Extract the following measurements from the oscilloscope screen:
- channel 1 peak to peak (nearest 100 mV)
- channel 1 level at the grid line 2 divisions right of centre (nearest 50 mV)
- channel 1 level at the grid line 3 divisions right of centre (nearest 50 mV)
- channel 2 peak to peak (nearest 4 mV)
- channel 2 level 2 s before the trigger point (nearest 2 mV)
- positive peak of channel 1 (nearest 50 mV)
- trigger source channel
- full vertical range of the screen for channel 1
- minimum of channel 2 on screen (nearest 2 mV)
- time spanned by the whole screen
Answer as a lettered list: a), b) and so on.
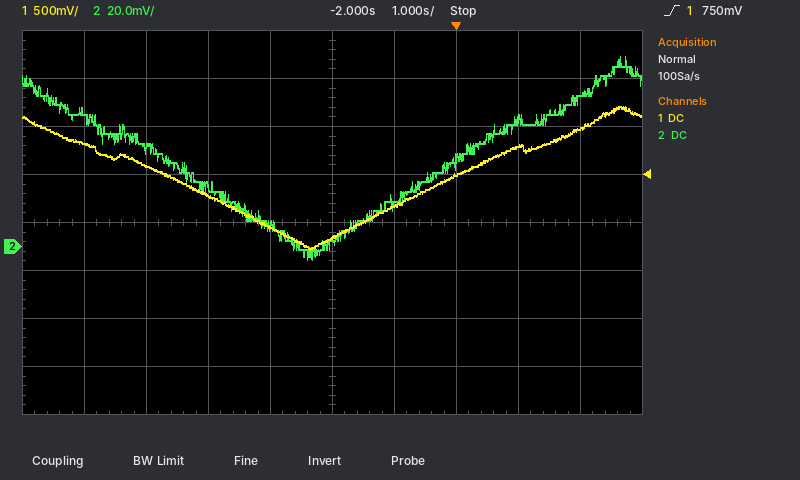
a) 1.50 V
b) 750 mV
c) 1.05 V
d) 84 mV
e) 0 mV
f) 1.45 V
g) channel 1
h) 4 V
i) -6 mV
j) 10 s
